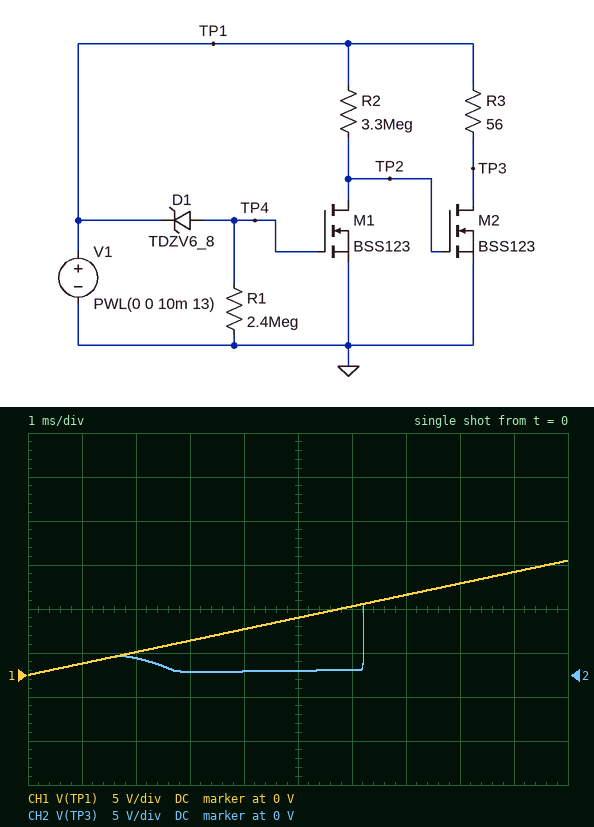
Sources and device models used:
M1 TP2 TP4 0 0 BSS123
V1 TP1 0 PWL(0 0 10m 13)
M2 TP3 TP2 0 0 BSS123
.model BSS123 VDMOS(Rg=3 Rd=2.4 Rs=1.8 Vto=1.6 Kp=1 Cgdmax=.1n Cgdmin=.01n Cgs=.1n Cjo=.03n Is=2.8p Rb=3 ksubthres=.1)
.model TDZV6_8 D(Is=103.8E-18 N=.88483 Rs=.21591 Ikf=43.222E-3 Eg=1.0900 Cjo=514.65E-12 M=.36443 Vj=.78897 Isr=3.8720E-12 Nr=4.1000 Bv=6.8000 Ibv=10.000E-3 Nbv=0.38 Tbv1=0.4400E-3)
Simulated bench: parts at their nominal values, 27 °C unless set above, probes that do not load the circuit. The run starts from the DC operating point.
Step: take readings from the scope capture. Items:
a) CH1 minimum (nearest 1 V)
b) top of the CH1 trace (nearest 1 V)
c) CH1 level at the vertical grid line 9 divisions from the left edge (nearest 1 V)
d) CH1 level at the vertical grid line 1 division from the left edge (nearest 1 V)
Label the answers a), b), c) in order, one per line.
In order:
a) 0 V
b) 13 V
c) 12 V
d) 1 V
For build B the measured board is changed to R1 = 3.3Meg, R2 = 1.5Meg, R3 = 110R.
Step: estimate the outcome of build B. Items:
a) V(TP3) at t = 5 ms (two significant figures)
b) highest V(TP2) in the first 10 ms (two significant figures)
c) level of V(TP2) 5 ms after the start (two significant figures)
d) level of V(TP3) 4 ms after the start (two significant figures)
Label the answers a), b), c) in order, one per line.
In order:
a) 6.5 V
b) 2.9 V
c) 1.3 V
d) 5.2 V
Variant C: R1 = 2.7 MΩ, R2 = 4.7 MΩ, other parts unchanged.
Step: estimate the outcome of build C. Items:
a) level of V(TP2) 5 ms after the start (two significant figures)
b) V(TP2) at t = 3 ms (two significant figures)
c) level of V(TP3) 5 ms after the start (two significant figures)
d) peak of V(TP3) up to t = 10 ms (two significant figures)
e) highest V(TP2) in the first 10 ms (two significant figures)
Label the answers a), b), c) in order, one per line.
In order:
a) 4.1 V
b) 1.6 V
c) 500 mV
d) 13 V
e) 5.9 V
